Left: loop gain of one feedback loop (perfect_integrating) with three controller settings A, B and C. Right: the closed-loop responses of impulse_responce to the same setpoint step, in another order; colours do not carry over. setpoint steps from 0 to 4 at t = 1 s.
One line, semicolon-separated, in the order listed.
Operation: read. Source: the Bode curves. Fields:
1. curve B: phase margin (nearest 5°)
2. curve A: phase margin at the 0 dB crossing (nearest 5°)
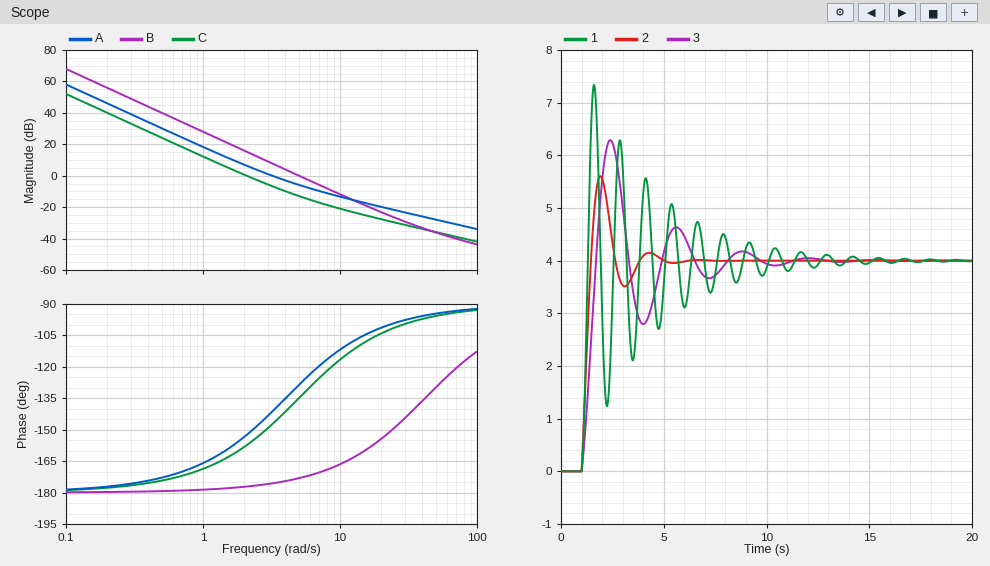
5°; 40°
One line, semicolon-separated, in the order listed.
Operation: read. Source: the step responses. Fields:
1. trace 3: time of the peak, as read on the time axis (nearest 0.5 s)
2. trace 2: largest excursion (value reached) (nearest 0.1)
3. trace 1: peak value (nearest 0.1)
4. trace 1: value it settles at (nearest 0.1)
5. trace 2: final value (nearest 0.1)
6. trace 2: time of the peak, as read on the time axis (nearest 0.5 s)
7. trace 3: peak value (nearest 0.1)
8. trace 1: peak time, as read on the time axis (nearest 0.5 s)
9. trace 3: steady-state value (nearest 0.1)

2.5 s; 5.6; 7.3; 4.0; 4.0; 2.0 s; 6.3; 1.5 s; 4.0
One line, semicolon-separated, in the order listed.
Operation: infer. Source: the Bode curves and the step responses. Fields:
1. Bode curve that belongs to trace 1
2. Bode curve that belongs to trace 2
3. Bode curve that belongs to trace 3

B; A; C
